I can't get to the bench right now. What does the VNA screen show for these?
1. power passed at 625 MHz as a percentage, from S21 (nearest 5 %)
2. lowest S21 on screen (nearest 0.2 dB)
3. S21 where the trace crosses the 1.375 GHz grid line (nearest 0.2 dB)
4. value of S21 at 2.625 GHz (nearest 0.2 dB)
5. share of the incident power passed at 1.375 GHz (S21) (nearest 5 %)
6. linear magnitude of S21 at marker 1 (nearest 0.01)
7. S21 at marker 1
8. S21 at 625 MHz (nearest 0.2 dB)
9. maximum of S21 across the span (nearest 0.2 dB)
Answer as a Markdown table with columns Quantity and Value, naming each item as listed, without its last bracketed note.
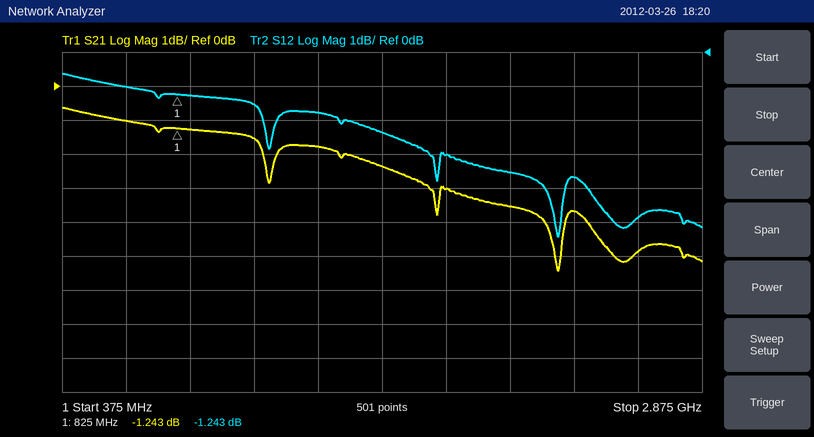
| Quantity | Value |
|---|---|
| power passed at 625 MHz as a percentage, from S21 | 80 % |
| lowest S21 on screen | -5.4 dB |
| S21 where the trace crosses the 1.375 GHz grid line | -1.8 dB |
| value of S21 at 2.625 GHz | -4.8 dB |
| share of the incident power passed at 1.375 GHz (S21) | 65 % |
| linear magnitude of S21 at marker 1 | 0.87 |
| S21 at marker 1 | -1.243 dB |
| S21 at 625 MHz | -1.0 dB |
| maximum of S21 across the span | -0.6 dB |
